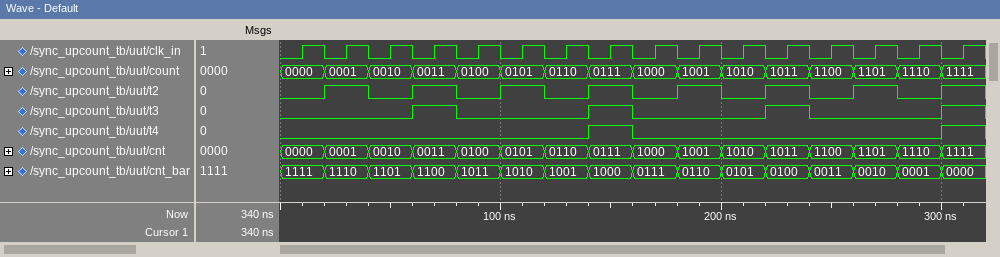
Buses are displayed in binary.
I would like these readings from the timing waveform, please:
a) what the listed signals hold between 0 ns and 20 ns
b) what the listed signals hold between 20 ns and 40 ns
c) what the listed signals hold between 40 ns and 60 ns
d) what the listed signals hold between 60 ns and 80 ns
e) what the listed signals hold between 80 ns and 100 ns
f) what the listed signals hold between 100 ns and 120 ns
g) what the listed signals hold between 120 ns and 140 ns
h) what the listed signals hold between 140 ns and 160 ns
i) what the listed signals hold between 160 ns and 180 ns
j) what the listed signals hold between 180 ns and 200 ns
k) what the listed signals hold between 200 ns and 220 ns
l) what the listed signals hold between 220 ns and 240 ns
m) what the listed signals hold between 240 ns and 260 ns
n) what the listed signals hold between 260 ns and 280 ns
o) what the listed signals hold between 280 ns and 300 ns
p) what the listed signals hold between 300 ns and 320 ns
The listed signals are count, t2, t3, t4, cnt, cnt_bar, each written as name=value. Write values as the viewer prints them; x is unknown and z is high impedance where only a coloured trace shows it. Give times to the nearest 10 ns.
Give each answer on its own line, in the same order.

count=0000, t2=0, t3=0, t4=0, cnt=0000, cnt_bar=1111
count=0001, t2=1, t3=0, t4=0, cnt=0001, cnt_bar=1110
count=0010, t2=0, t3=0, t4=0, cnt=0010, cnt_bar=1101
count=0011, t2=1, t3=1, t4=0, cnt=0011, cnt_bar=1100
count=0100, t2=0, t3=0, t4=0, cnt=0100, cnt_bar=1011
count=0101, t2=1, t3=0, t4=0, cnt=0101, cnt_bar=1010
count=0110, t2=0, t3=0, t4=0, cnt=0110, cnt_bar=1001
count=0111, t2=1, t3=1, t4=1, cnt=0111, cnt_bar=1000
count=1000, t2=0, t3=0, t4=0, cnt=1000, cnt_bar=0111
count=1001, t2=1, t3=0, t4=0, cnt=1001, cnt_bar=0110
count=1010, t2=0, t3=0, t4=0, cnt=1010, cnt_bar=0101
count=1011, t2=1, t3=1, t4=0, cnt=1011, cnt_bar=0100
count=1100, t2=0, t3=0, t4=0, cnt=1100, cnt_bar=0011
count=1101, t2=1, t3=0, t4=0, cnt=1101, cnt_bar=0010
count=1110, t2=0, t3=0, t4=0, cnt=1110, cnt_bar=0001
count=1111, t2=1, t3=1, t4=1, cnt=1111, cnt_bar=0000
